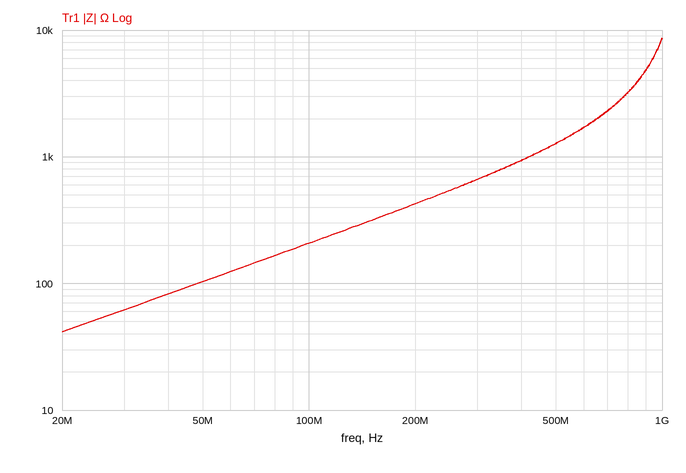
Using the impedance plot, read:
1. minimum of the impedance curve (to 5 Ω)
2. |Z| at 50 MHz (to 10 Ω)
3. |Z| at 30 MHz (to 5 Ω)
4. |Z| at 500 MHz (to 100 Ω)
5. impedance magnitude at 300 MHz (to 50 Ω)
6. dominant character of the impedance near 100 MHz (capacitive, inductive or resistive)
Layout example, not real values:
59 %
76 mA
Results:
40 Ω
100 Ω
60 Ω
1.3 kΩ
650 Ω
inductive
